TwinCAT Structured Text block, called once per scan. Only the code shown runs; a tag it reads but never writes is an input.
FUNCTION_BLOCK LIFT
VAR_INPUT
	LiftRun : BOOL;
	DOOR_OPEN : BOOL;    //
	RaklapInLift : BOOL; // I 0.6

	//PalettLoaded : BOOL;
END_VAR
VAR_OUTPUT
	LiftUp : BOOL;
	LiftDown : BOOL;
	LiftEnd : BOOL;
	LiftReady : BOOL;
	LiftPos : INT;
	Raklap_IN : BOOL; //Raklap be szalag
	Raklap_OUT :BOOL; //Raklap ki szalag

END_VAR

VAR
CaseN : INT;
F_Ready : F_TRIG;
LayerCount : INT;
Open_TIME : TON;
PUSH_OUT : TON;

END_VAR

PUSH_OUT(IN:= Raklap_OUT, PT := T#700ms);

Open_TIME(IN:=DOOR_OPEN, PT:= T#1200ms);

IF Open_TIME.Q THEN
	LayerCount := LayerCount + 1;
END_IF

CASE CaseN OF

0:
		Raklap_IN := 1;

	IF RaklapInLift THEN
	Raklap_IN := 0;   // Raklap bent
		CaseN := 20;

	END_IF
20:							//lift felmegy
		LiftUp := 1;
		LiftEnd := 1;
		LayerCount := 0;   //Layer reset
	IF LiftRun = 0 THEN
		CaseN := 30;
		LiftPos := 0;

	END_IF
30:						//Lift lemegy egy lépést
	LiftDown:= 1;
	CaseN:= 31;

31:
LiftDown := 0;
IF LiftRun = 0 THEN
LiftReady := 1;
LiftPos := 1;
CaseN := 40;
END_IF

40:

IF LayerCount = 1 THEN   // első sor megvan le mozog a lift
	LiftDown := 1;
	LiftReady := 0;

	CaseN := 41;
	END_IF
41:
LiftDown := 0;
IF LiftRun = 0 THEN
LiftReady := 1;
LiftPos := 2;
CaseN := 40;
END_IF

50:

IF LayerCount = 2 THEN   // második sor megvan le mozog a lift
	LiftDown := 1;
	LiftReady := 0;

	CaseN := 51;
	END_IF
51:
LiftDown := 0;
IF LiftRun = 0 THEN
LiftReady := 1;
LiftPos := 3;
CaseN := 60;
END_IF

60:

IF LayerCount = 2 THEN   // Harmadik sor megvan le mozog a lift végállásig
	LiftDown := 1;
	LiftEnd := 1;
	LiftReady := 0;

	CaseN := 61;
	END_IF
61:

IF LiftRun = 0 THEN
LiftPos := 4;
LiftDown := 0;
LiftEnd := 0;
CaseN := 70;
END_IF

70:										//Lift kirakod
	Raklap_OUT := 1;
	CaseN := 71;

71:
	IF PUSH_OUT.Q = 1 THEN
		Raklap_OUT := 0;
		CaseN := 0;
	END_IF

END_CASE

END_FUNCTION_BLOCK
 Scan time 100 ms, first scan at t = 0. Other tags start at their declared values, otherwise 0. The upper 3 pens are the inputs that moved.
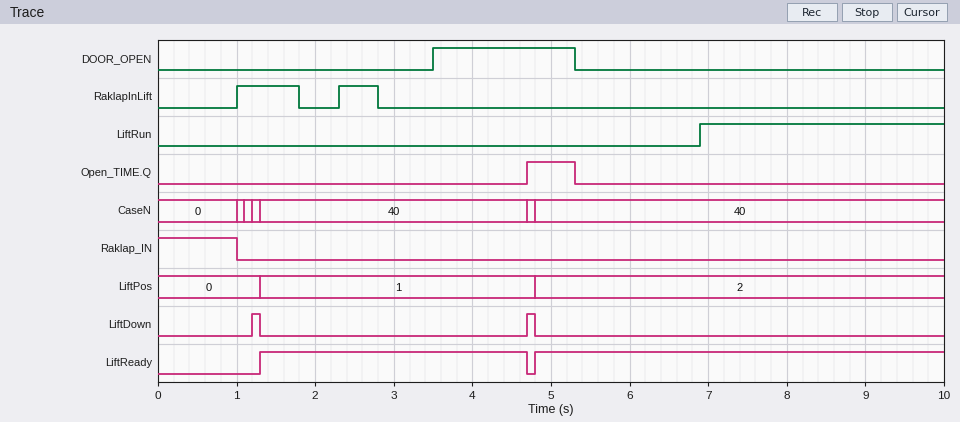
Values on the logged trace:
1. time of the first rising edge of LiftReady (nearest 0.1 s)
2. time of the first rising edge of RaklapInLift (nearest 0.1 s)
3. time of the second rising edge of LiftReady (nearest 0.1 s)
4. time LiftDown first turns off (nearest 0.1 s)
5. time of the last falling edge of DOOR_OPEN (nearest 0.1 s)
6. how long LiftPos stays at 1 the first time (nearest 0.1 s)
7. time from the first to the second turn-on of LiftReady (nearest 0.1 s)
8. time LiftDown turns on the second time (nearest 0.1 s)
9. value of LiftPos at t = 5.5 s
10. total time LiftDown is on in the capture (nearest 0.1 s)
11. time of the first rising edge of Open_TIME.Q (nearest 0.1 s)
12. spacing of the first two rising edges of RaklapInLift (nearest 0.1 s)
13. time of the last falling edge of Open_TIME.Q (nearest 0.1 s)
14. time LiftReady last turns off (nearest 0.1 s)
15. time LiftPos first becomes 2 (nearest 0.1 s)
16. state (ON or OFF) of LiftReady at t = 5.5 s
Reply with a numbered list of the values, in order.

1. 1.3 s
2. 1.0 s
3. 4.8 s
4. 1.3 s
5. 5.3 s
6. 3.5 s
7. 3.5 s
8. 4.7 s
9. 2
10. 0.2 s
11. 4.7 s
12. 1.3 s
13. 5.3 s
14. 4.7 s
15. 4.8 s
16. ON
